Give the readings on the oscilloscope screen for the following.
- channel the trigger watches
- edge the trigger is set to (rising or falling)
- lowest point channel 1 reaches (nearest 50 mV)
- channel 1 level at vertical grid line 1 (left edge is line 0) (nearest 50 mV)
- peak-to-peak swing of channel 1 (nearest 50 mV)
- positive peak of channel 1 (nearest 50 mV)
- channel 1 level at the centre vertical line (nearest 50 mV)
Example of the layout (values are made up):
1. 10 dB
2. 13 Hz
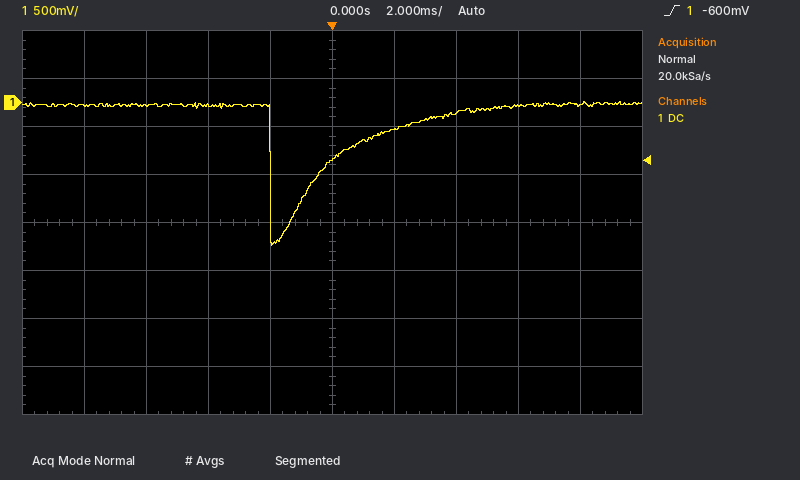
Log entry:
1. channel 1
2. rising
3. -1.50 V
4. -50 mV
5. 1.50 V
6. 0 mV
7. -600 mV
